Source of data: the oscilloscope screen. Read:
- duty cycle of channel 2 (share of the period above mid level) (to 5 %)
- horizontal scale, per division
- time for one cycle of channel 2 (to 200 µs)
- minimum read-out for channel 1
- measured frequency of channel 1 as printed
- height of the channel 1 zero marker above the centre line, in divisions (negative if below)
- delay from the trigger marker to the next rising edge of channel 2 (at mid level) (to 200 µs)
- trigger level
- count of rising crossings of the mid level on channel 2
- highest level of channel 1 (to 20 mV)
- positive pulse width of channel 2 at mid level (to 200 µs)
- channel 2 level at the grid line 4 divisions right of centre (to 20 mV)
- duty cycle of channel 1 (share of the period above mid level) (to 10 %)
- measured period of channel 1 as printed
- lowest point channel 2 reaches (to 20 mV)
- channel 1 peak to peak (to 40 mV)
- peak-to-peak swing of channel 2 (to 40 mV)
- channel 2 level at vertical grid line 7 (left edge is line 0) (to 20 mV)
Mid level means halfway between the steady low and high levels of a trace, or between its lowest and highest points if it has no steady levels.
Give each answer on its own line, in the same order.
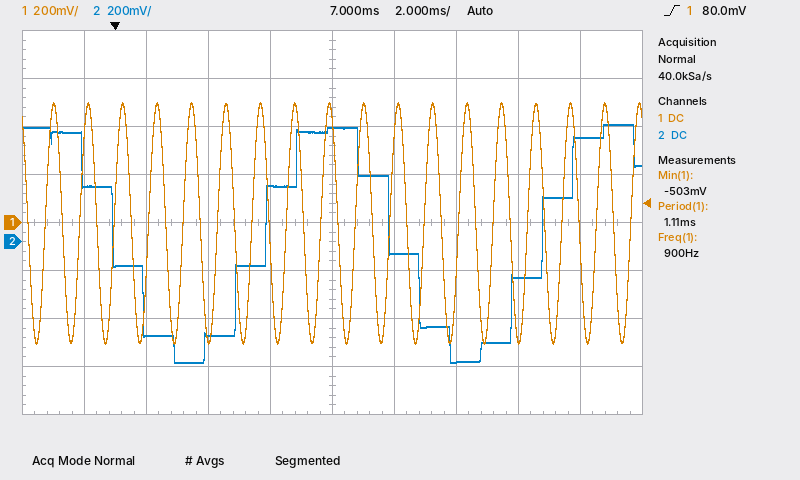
45 %
2 ms
9.0 ms
-503 mV
900 Hz
0.0 div
4.8 ms
80.0 mV
2
500 mV
4.0 ms
440 mV
50 %
1.11 ms
-500 mV
1.00 V
1.00 V
-500 mV
